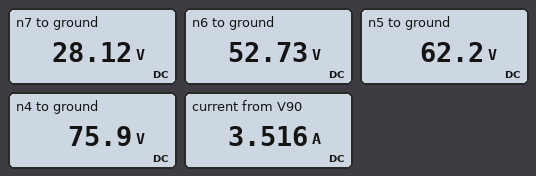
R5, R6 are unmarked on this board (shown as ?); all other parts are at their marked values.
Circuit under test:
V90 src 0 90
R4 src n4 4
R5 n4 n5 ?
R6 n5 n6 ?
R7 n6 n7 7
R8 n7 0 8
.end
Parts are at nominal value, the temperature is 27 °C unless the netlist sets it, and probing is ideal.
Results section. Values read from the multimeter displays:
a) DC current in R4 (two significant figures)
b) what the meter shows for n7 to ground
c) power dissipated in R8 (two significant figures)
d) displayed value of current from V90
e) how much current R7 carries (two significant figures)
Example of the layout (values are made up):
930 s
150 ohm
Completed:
3.5 A
28.12 V
99 W
3.516 A
3.5 A
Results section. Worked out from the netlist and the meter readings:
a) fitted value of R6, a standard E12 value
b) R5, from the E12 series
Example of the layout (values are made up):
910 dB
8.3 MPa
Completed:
2.7 Ω
3.9 Ω
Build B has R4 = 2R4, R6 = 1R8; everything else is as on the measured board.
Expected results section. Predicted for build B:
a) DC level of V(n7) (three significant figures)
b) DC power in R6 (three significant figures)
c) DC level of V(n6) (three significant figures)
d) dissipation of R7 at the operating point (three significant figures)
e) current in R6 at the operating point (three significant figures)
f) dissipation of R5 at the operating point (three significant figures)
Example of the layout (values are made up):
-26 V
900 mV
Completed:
31.2 V
27.3 W
58.4 V
106 W
3.90 A
59.2 W
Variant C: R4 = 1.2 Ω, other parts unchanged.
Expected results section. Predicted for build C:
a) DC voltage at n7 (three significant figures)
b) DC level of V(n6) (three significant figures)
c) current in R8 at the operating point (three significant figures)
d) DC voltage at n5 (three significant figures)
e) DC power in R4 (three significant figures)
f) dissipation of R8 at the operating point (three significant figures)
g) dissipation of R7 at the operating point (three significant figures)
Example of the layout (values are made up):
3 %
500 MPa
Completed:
31.6 V
59.2 V
3.95 A
69.9 V
18.7 W
125 W
109 W
